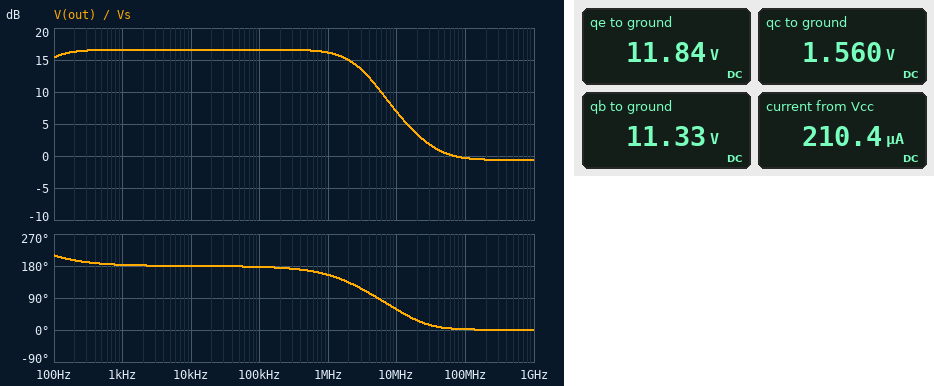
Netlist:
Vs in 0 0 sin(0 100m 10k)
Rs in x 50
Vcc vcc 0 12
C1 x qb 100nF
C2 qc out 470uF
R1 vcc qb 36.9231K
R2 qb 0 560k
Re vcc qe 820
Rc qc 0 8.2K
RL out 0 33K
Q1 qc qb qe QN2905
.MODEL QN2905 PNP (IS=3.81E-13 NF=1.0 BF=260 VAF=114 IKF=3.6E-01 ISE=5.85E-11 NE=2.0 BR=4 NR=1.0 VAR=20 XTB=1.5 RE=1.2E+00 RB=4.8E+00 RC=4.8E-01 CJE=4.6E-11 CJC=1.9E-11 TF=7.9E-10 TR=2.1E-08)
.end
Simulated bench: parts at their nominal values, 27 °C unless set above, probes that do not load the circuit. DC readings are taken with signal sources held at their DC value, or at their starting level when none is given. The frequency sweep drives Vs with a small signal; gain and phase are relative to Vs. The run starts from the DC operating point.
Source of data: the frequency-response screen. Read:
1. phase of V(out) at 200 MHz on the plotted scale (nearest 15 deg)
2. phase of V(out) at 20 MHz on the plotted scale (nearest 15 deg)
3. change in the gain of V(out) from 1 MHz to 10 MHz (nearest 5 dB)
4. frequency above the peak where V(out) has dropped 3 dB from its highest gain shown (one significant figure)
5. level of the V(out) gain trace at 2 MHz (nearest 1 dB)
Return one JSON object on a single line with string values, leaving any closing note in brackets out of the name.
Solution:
{"phase of V(out) at 200 MHz on the plotted scale": "0 deg", "phase of V(out) at 20 MHz on the plotted scale": "30 deg", "change in the gain of V(out) from 1 MHz to 10 MHz": "-10 dB", "frequency above the peak where V(out) has dropped 3 dB from its highest gain shown": "3 MHz", "level of the V(out) gain trace at 2 MHz": "15 dB"}
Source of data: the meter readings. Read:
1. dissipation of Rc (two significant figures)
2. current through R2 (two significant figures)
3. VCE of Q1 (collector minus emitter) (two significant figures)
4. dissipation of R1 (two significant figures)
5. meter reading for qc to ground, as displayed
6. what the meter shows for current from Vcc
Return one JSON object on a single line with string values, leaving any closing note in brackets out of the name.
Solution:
{"dissipation of Rc": "300 µW", "current through R2": "20 µA", "VCE of Q1 (collector minus emitter)": "-10 V", "dissipation of R1": "12 µW", "meter reading for qc to ground, as displayed": "1.560 V", "what the meter shows for current from Vcc": "210.4 µA"}
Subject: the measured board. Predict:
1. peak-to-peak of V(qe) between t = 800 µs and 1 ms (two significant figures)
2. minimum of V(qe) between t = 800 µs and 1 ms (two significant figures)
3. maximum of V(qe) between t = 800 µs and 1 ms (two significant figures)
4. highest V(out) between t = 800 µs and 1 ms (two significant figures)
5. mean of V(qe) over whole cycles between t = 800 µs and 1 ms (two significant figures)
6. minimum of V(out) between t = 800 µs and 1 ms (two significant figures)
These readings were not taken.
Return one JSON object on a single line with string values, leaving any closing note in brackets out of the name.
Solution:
{"peak-to-peak of V(qe) between t = 800 µs and 1 ms": "170 mV", "minimum of V(qe) between t = 800 µs and 1 ms": "12 V", "maximum of V(qe) between t = 800 µs and 1 ms": "12 V", "highest V(out) between t = 800 µs and 1 ms": "700 mV", "mean of V(qe) over whole cycles between t = 800 µs and 1 ms": "12 V", "minimum of V(out) between t = 800 µs and 1 ms": "-640 mV"}
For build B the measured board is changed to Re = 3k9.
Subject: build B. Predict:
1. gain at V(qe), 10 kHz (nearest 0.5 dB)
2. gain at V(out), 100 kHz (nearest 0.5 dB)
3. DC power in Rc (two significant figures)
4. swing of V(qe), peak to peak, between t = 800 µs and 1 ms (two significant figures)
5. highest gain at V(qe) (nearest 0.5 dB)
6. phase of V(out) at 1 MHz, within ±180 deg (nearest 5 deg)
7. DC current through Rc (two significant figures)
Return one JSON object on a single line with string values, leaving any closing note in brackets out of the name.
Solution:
{"gain at V(qe), 10 kHz": "-1.0 dB", "gain at V(out), 100 kHz": "3.5 dB", "DC power in Rc": "27 µW", "swing of V(qe), peak to peak, between t = 800 µs and 1 ms": "180 mV", "highest gain at V(qe)": "0 dB", "phase of V(out) at 1 MHz, within ±180 deg": "140 deg", "DC current through Rc": "57 µA"}
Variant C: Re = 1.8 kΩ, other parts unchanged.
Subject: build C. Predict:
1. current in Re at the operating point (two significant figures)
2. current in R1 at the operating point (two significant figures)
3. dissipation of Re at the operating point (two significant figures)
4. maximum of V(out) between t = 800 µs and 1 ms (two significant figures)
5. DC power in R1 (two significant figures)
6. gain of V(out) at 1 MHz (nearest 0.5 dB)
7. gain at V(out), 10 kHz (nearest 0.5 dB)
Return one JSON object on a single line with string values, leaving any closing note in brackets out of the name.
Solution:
{"current in Re at the operating point": "110 µA", "current in R1 at the operating point": "19 µA", "dissipation of Re at the operating point": "21 µW", "maximum of V(out) between t = 800 µs and 1 ms": "330 mV", "DC power in R1": "13 µW", "gain of V(out) at 1 MHz": "9.5 dB", "gain at V(out), 10 kHz": "10.0 dB"}
